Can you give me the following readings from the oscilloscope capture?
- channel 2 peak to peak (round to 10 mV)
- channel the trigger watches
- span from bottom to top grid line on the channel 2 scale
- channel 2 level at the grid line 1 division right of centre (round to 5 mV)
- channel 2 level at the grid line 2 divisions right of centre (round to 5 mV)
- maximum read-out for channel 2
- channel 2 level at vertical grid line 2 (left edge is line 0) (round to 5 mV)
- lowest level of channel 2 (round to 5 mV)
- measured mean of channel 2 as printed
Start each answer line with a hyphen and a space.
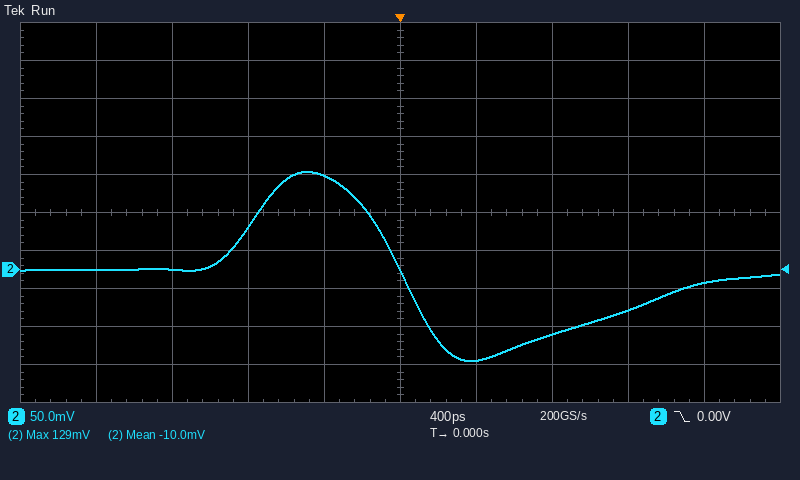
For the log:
- 250 mV
- channel 2
- 500 mV
- -120 mV
- -85 mV
- 129 mV
- 0 mV
- -120 mV
- -10.0 mV
